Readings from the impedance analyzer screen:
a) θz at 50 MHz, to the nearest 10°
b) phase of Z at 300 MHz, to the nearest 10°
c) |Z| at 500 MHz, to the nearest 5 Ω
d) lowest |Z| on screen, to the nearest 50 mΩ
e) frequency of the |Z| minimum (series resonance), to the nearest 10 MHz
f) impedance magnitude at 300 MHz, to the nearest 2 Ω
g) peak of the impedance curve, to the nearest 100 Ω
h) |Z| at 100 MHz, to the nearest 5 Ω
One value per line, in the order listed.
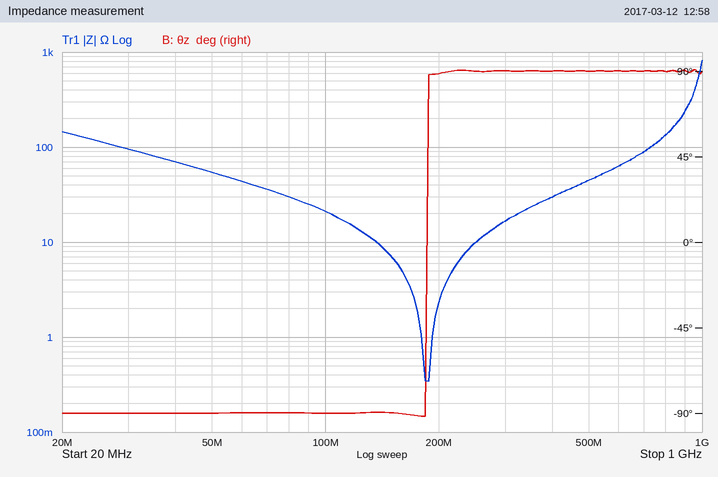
-90°
90°
45 Ω
350 mΩ
190 MHz
16 Ω
800 Ω
20 Ω
